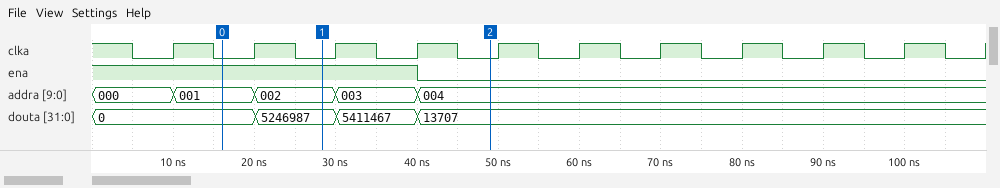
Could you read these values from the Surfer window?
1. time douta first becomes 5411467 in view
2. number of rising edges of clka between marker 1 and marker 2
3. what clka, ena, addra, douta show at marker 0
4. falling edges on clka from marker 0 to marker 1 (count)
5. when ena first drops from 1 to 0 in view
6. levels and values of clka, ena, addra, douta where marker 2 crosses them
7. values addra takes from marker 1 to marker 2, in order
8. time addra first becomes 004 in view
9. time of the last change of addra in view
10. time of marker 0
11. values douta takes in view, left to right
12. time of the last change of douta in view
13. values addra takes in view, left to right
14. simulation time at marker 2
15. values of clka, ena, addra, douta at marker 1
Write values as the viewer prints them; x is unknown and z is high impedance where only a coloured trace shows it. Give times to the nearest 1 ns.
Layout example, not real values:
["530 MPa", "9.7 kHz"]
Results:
["30 ns", "2", "clka=0, ena=1, addra=001, douta=0", "1", "40 ns", "clka=0, ena=0, addra=004, douta=13707", "002, 003, 004", "40 ns", "40 ns", "16 ns", "0, 5246987, 5411467, 13707", "40 ns", "000, 001, 002, 003, 004", "49 ns", "clka=0, ena=1, addra=002, douta=5246987"]
